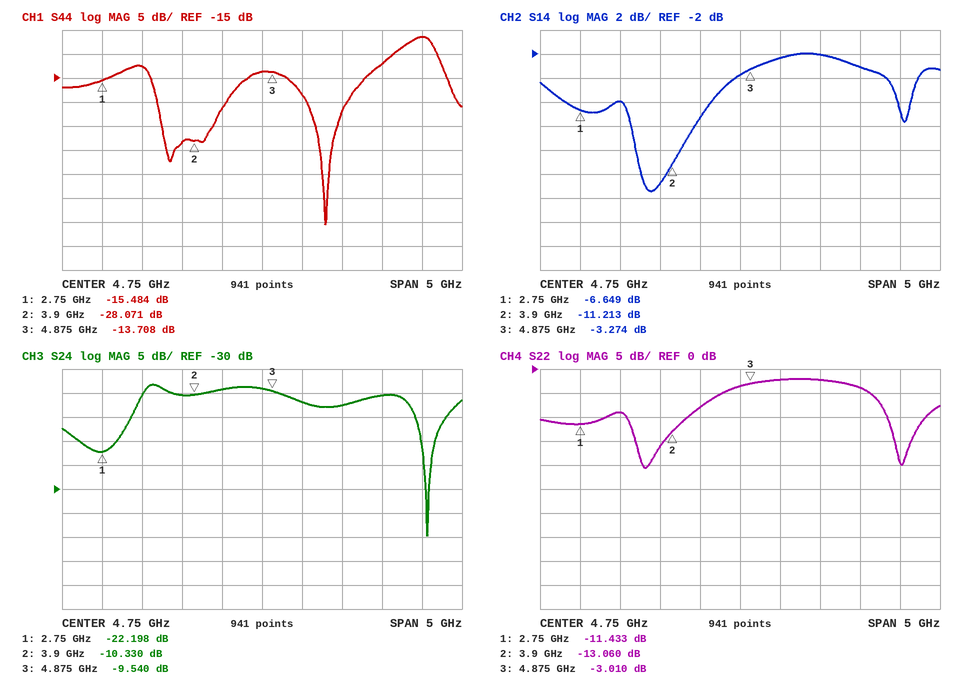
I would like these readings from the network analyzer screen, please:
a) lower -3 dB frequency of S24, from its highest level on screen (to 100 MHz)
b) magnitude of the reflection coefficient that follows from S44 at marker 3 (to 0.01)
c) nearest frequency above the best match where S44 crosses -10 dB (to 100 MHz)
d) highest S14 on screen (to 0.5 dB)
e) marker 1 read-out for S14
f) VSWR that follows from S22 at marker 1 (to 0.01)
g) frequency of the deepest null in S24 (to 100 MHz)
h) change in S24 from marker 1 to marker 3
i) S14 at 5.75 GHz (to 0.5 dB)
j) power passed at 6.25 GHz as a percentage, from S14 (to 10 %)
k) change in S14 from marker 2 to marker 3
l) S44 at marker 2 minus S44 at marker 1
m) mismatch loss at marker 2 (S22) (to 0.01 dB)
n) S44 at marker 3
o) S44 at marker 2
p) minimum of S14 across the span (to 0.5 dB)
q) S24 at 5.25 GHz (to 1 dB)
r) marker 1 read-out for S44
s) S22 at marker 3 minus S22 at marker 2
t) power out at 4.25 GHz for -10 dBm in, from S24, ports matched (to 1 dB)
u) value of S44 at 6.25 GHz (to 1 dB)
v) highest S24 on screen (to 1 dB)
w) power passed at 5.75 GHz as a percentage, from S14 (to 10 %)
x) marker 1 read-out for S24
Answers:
3.2 GHz
0.21
6.4 GHz
-2.0 dB
-6.649 dB
1.73
6.8 GHz
12.658 dB
-2.0 dB
50 %
7.939 dB
-12.587 dB
0.22 dB
-13.708 dB
-28.071 dB
-13.5 dB
-12 dB
-15.484 dB
10.050 dB
-19 dBm
-12 dB
-8 dB
60 %
-22.198 dB
